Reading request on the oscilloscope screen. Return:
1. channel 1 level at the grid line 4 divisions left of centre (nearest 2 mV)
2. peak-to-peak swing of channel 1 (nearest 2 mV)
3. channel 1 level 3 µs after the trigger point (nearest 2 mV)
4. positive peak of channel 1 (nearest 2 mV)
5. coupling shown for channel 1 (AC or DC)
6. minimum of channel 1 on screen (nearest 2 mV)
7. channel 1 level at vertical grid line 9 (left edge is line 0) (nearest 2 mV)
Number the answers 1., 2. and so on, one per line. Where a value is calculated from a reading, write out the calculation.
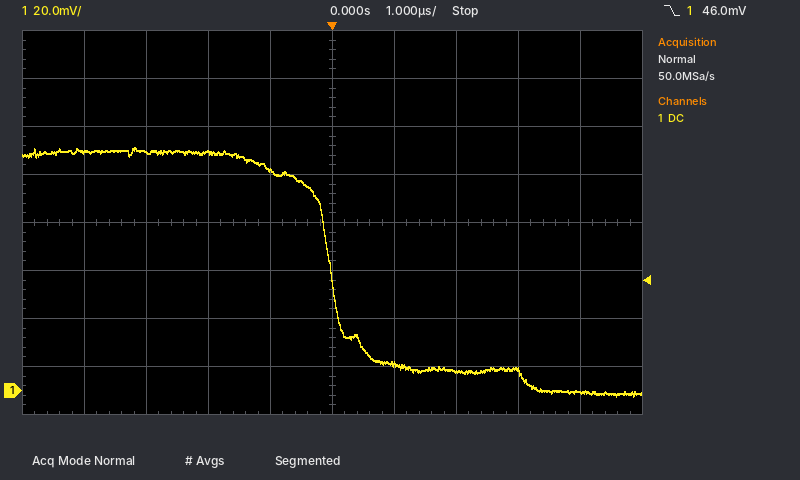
1. 100 mV
2. 102 mV − (-2 mV) = 104 mV
3. 8 mV
4. 102 mV
5. DC
6. -2 mV
7. 0 mV
